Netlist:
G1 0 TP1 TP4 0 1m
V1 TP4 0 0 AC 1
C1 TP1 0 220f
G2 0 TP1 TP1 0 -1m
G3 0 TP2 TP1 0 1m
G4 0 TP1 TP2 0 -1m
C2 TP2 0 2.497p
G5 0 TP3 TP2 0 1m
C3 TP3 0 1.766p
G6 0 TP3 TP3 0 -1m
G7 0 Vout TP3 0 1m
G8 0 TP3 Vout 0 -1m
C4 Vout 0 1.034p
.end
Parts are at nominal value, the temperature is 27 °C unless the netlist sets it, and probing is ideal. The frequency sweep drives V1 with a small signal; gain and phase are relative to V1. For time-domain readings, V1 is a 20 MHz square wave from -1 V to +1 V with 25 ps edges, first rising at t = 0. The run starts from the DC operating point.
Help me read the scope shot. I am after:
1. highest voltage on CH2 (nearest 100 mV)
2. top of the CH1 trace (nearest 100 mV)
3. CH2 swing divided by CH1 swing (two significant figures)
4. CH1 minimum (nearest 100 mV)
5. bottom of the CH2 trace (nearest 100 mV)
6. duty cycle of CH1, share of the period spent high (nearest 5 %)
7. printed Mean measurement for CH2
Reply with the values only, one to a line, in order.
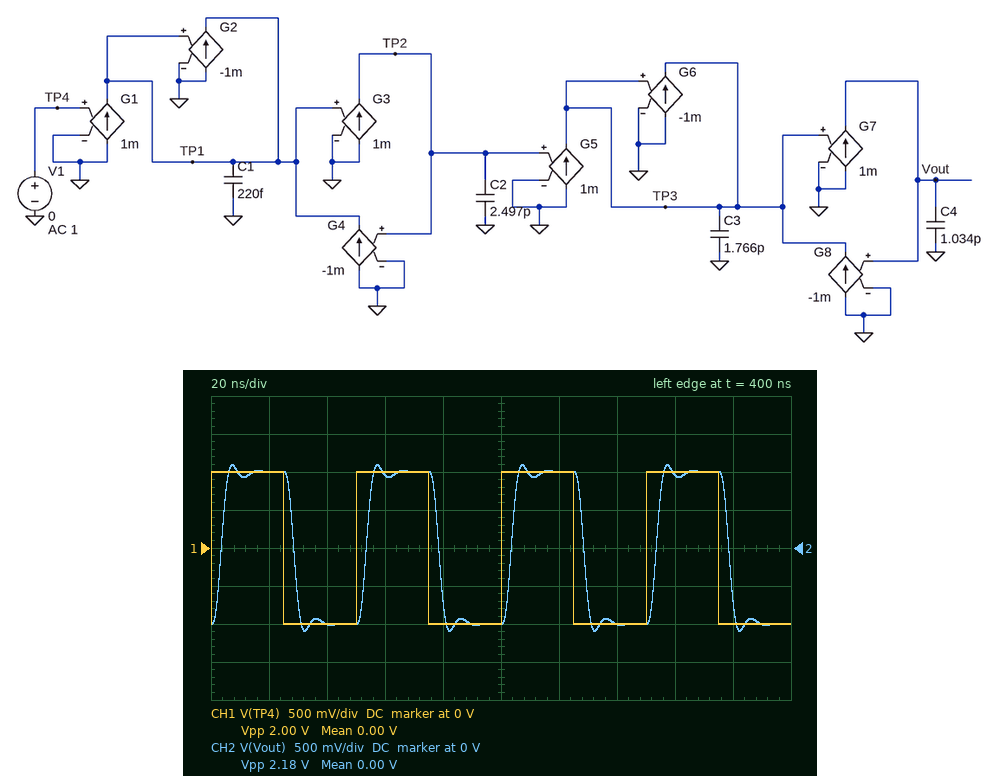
1.1 V
1.0 V
1.1
-1.0 V
-1.1 V
50 %
0.00 V
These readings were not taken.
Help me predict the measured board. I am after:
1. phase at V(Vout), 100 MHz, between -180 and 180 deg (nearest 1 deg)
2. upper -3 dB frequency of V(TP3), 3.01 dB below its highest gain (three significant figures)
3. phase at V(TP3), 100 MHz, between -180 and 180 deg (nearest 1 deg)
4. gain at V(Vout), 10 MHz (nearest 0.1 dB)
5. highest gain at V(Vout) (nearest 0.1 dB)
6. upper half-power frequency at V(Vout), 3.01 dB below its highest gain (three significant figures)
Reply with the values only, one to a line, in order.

-130 deg
145 MHz
-40 deg
0 dB
0 dB
113 MHz
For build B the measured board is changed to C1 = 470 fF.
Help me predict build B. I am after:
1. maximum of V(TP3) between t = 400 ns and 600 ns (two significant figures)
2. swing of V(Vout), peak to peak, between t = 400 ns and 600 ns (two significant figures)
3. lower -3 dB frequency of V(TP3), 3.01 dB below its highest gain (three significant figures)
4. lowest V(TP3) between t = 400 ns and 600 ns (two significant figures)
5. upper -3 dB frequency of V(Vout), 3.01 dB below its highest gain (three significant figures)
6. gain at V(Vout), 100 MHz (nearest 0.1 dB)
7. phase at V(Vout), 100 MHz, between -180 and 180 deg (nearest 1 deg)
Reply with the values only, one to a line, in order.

580 mV
2.3 V
64.0 MHz
-580 mV
117 MHz
-1.4 dB
-138 deg
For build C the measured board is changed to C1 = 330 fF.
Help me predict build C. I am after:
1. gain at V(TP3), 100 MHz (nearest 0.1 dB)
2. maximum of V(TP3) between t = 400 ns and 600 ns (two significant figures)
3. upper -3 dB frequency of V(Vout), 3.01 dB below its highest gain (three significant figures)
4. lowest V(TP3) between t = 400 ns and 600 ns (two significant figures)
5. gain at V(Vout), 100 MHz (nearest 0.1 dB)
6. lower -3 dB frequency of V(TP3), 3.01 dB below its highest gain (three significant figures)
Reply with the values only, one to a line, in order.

-5.4 dB
570 mV
115 MHz
-570 mV
-1.6 dB
64.0 MHz
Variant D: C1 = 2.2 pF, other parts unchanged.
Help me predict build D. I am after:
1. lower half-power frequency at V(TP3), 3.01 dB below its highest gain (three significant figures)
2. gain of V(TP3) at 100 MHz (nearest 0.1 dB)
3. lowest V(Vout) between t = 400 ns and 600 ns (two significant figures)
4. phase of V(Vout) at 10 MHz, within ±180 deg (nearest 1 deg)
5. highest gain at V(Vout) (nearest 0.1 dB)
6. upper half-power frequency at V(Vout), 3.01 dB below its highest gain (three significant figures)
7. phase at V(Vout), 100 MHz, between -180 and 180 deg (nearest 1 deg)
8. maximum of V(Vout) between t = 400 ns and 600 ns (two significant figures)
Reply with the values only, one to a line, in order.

46.6 MHz
-6.6 dB
-1.5 V
-13 deg
2.0 dB
88.9 MHz
167 deg
1.5 V
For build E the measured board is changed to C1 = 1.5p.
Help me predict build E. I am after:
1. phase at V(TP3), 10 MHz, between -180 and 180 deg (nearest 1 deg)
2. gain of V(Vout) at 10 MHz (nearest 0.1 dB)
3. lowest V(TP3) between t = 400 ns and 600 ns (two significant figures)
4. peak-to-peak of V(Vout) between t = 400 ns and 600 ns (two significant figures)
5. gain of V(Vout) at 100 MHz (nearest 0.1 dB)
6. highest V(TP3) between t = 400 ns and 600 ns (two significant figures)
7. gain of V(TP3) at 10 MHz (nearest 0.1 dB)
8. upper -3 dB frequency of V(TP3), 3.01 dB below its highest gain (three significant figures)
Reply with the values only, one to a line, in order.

77 deg
0.1 dB
-570 mV
2.8 V
-1.3 dB
570 mV
-23.7 dB
127 MHz
